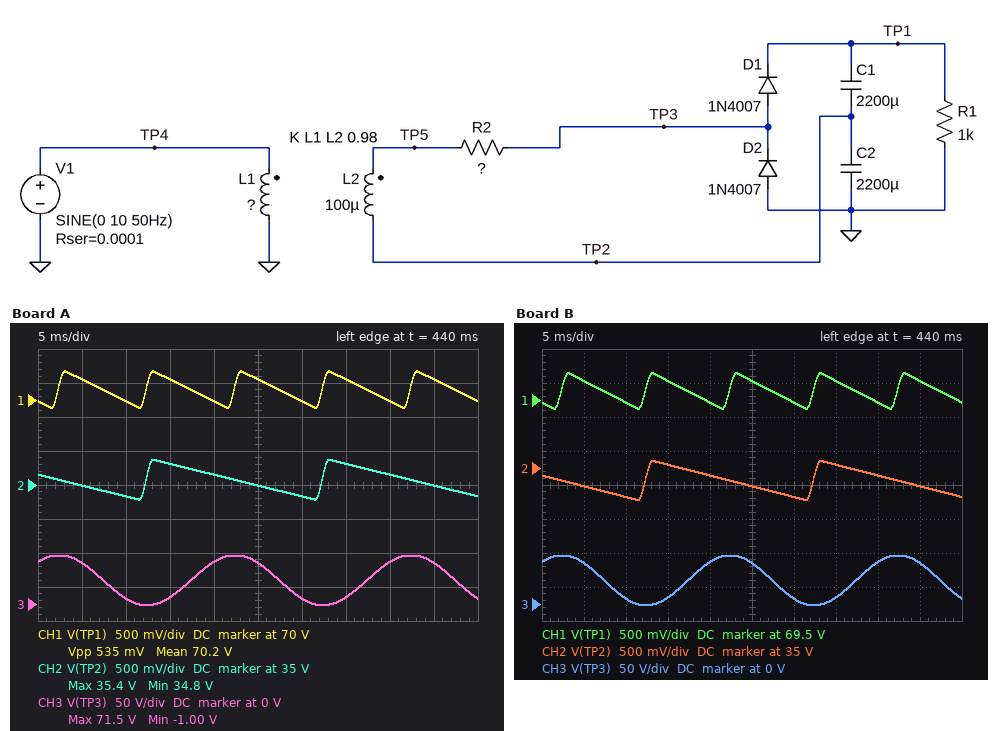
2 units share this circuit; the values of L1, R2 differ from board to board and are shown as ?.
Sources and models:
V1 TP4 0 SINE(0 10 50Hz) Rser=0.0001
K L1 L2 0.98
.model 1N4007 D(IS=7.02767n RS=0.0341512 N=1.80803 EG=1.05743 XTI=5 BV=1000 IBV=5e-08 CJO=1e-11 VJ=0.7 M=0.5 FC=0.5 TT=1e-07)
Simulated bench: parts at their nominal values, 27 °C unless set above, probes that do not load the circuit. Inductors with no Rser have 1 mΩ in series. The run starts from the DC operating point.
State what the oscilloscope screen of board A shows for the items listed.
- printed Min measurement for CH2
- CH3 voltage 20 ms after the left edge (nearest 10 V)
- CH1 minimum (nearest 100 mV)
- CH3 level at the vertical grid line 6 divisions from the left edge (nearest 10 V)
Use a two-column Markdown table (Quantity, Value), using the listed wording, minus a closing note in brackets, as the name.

| Quantity | Value |
|---|---|
| printed Min measurement for CH2 | 34.8 V |
| CH3 voltage 20 ms after the left edge | 60 V |
| CH1 minimum | 69.9 V |
| CH3 level at the vertical grid line 6 divisions from the left edge | 10 V |
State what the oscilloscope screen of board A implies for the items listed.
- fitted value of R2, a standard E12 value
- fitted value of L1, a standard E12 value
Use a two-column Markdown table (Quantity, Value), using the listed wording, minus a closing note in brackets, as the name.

| Quantity | Value |
|---|---|
| fitted value of R2, a standard E12 value | 0.68 Ω |
| fitted value of L1, a standard E12 value | 3.3 µH |
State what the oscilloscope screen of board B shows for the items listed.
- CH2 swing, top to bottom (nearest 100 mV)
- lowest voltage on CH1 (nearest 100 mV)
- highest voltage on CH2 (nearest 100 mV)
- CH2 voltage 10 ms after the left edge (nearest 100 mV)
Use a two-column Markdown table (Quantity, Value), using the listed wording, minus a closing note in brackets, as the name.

| Quantity | Value |
|---|---|
| CH2 swing, top to bottom | 600 mV |
| lowest voltage on CH1 | 69.4 V |
| highest voltage on CH2 | 35.1 V |
| CH2 voltage 10 ms after the left edge | 34.6 V |
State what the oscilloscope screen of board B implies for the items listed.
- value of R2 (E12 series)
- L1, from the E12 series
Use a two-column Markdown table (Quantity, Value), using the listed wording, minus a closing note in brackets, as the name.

| Quantity | Value |
|---|---|
| value of R2 | 1 Ω |
| L1, from the E12 series | 3.3 µH |
